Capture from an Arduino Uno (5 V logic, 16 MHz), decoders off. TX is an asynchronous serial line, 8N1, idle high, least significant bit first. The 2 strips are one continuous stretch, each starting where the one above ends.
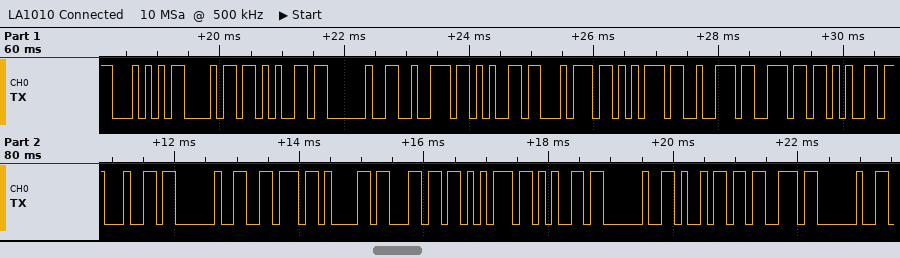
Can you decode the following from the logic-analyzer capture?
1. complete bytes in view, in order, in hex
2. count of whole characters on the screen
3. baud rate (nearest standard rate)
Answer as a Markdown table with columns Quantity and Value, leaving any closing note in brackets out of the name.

| Quantity | Value |
|---|---|
| complete bytes in view, in order, in hex | 54 68 65 20 72 65 74 75 72 6E 65 64 20 76 61 6C 75 65 20 69 73 20 |
| count of whole characters on the screen | 22 |
| baud rate | 9600 baud |
